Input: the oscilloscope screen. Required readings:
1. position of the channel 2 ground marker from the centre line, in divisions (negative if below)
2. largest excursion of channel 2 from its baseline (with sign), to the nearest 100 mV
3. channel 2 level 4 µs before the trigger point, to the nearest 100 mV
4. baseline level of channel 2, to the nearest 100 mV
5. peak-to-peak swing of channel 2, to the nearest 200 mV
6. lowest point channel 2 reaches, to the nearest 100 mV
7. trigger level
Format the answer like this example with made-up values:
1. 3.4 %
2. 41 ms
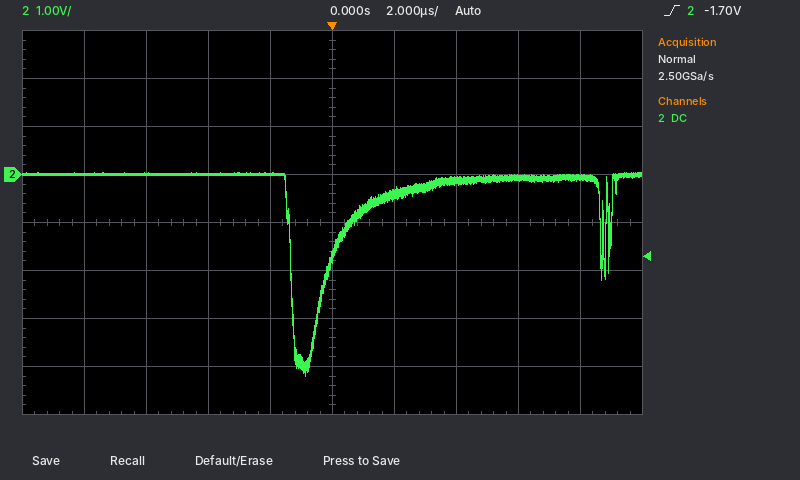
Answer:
1. +1.0 div
2. -4.2 V
3. 0.0 V
4. 0.0 V
5. 4.2 V
6. -4.2 V
7. -1.70 V
